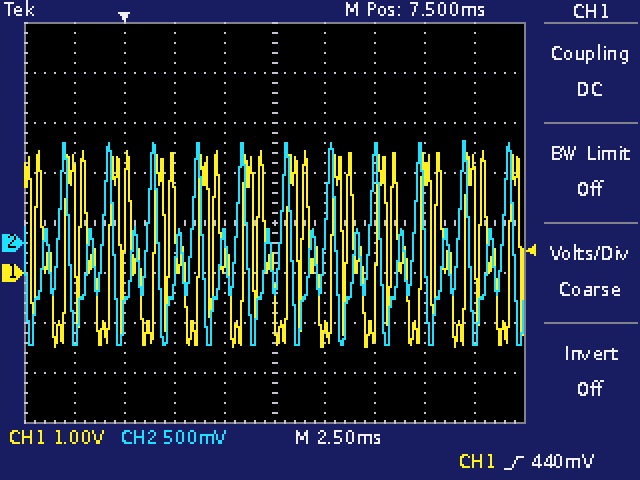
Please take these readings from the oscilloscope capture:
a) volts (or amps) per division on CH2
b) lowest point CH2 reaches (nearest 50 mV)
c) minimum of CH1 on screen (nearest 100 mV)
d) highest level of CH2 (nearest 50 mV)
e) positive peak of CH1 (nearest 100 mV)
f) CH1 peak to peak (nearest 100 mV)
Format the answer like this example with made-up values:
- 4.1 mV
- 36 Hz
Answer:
- 500 mV
- -1.00 V
- -1.5 V
- 1.00 V
- 2.4 V
- 3.9 V
